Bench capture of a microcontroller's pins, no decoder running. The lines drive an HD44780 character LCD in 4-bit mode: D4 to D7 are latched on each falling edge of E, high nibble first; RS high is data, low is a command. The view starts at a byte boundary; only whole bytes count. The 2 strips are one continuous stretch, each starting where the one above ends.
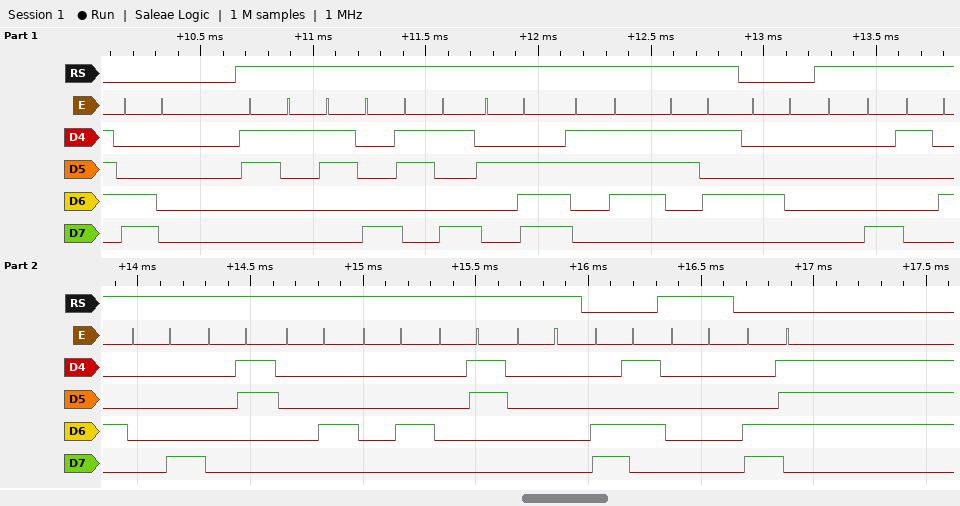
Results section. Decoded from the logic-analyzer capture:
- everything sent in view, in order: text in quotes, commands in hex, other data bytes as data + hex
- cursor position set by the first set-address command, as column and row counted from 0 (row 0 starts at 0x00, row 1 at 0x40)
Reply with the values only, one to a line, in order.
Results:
0xC0 "189.75" 0x40 data 08 14 08 03 04 04 03 00 0xC5 data 00 0xC7
column 0, row 1
